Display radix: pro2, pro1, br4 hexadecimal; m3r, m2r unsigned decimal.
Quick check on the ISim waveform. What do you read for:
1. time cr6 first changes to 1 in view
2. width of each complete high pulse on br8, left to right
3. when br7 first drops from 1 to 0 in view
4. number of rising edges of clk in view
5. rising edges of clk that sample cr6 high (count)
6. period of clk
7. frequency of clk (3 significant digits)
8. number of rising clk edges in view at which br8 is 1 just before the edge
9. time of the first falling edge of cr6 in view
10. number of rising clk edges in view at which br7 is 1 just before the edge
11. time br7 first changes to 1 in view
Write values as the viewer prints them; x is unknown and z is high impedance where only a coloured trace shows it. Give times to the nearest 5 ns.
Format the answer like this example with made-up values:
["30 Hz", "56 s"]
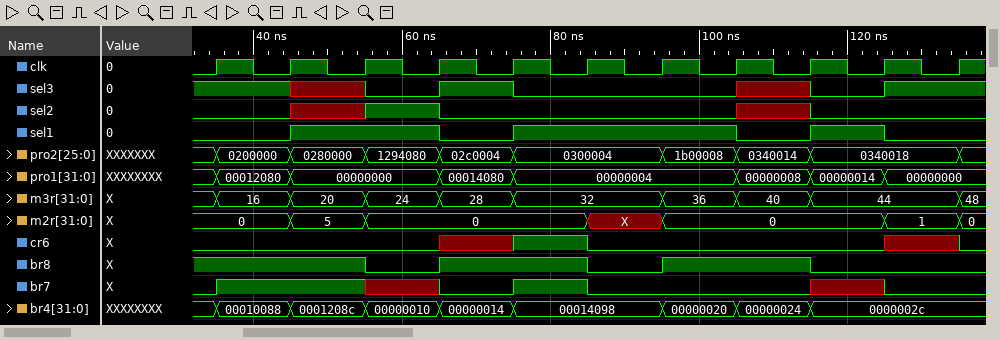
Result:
["75 ns", "20 ns, 20 ns", "85 ns", "11", "1", "10 ns", "100 MHz", "7", "85 ns", "3", "35 ns"]
